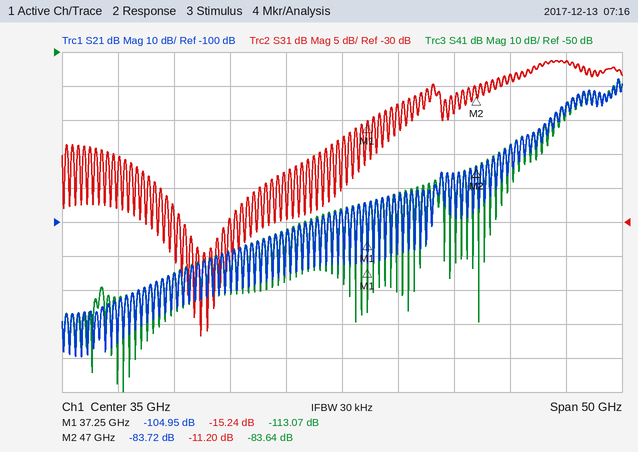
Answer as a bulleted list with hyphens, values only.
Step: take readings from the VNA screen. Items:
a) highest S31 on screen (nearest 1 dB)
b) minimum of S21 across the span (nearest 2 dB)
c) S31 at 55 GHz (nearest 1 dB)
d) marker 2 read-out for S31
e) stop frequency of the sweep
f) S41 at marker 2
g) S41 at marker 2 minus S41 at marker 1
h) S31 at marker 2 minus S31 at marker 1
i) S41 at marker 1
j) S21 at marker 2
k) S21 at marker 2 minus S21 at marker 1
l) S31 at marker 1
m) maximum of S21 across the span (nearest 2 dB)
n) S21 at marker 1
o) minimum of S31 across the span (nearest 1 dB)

- -6 dB
- -140 dB
- -6 dB
- -11.20 dB
- 60 GHz
- -83.64 dB
- 29.43 dB
- 4.04 dB
- -113.07 dB
- -83.72 dB
- 21.23 dB
- -15.24 dB
- -58 dB
- -104.95 dB
- -47 dB
